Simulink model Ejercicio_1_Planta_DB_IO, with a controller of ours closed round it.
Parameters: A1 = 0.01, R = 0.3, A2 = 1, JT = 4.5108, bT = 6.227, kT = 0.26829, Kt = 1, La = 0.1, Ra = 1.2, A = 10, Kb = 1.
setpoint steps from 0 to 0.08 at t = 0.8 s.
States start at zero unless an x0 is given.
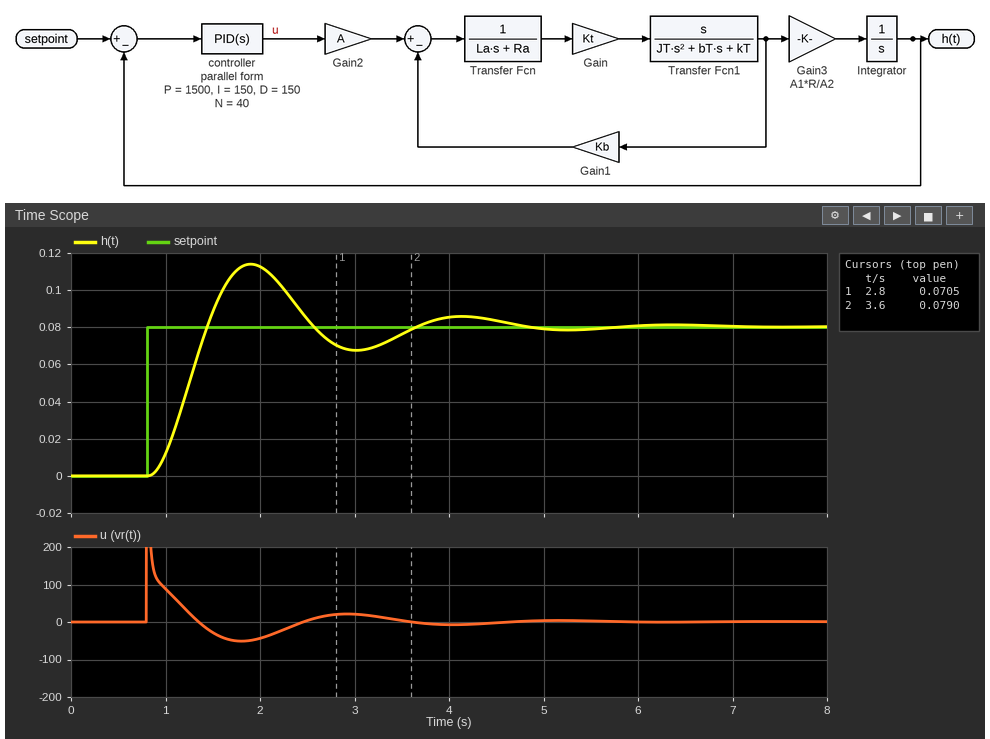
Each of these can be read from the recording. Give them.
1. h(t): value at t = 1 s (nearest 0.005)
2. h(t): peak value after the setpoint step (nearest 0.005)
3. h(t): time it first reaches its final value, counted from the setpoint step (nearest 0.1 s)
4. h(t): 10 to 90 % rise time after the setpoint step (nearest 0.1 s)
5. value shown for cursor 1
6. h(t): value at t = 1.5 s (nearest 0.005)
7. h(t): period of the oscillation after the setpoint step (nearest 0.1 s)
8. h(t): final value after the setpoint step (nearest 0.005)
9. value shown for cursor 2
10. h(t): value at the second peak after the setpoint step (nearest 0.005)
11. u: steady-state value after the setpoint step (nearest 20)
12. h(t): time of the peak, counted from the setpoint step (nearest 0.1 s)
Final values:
0.010
0.115
0.6 s
0.4 s
0.0705
0.090
2.2 s
0.080
0.0790
0.085
0
1.1 s
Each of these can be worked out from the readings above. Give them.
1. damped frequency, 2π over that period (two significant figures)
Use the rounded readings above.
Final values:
2.9 rad/s
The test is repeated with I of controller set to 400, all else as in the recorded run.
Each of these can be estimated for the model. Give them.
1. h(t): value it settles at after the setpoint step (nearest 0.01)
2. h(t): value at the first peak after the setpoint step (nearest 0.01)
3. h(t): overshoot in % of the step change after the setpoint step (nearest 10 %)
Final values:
0.08
0.12
50 %
